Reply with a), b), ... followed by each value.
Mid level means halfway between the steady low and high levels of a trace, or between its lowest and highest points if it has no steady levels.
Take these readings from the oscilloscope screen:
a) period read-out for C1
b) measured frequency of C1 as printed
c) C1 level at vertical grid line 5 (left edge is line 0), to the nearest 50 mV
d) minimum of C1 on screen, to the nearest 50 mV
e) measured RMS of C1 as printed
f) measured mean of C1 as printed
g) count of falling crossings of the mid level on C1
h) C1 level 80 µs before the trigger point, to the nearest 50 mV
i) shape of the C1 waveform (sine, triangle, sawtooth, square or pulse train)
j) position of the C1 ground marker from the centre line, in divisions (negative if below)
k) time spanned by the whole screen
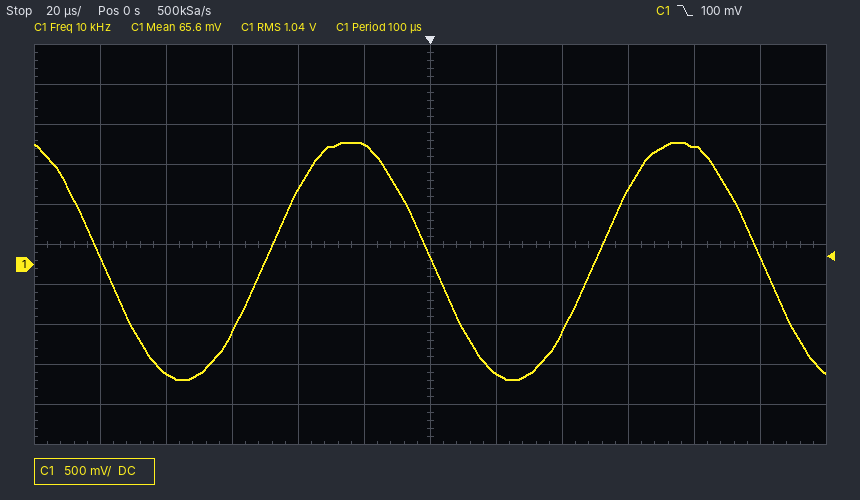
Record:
a) 100 µs
b) 10 kHz
c) 1.50 V
d) -1.45 V
e) 1.04 V
f) 65.6 mV
g) 3
h) -1.35 V
i) sine
j) -0.5 div
k) 240 µs
